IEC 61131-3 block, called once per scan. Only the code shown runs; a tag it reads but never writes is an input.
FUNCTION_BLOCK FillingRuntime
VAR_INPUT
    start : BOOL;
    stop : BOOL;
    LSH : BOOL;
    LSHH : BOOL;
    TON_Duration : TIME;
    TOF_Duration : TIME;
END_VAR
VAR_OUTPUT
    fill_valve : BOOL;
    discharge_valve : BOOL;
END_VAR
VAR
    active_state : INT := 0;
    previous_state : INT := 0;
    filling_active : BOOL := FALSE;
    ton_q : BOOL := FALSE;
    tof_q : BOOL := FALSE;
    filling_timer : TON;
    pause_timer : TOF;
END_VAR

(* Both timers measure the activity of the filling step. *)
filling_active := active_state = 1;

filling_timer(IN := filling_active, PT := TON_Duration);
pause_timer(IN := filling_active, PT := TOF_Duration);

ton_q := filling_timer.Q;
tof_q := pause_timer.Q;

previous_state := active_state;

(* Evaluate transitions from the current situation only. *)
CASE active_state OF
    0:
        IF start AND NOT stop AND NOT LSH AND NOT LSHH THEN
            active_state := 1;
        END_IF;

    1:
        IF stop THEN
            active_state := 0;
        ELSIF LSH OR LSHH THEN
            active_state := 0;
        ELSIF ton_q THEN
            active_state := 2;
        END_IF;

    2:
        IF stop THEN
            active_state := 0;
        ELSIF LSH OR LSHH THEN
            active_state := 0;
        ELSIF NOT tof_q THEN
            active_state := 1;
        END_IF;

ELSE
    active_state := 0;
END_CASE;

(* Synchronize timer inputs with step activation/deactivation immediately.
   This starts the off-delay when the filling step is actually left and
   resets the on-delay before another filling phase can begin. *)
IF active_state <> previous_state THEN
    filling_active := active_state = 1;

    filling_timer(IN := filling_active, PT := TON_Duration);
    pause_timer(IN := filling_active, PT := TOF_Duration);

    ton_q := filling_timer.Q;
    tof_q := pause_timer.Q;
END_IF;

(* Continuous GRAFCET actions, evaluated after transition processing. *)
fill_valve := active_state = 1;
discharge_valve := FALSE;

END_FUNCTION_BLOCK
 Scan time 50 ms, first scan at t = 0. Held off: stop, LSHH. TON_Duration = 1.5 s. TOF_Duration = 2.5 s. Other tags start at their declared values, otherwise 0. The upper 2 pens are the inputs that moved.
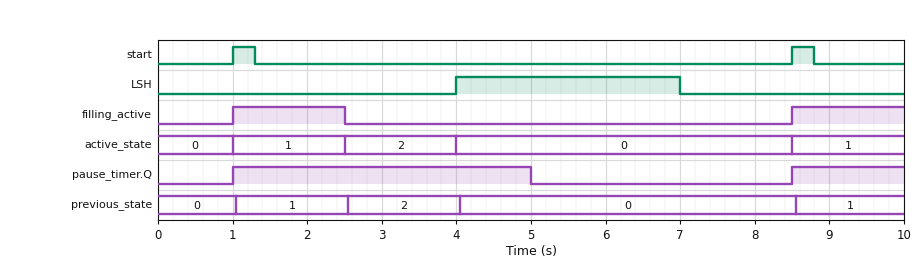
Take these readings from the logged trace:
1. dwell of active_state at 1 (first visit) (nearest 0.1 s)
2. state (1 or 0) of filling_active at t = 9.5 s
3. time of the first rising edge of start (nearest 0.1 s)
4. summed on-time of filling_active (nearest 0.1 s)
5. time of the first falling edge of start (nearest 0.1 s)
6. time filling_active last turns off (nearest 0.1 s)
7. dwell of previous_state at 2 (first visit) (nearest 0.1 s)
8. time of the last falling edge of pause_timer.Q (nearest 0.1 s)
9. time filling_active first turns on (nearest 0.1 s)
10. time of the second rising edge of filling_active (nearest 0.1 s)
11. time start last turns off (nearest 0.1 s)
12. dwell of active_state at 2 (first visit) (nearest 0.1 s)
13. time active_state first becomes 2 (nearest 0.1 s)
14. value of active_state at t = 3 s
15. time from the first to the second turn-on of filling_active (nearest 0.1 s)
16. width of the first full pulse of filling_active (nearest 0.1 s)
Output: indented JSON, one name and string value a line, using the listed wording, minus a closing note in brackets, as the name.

{
  "dwell of active_state at 1 (first visit)": "1.5 s",
  "state (1 or 0) of filling_active at t = 9.5 s": "1",
  "time of the first rising edge of start": "1.0 s",
  "summed on-time of filling_active": "3.0 s",
  "time of the first falling edge of start": "1.3 s",
  "time filling_active last turns off": "2.5 s",
  "dwell of previous_state at 2 (first visit)": "1.5 s",
  "time of the last falling edge of pause_timer.Q": "5.0 s",
  "time filling_active first turns on": "1.0 s",
  "time of the second rising edge of filling_active": "8.5 s",
  "time start last turns off": "8.8 s",
  "dwell of active_state at 2 (first visit)": "1.5 s",
  "time active_state first becomes 2": "2.5 s",
  "value of active_state at t = 3 s": "2",
  "time from the first to the second turn-on of filling_active": "7.5 s",
  "width of the first full pulse of filling_active": "1.5 s"
}
